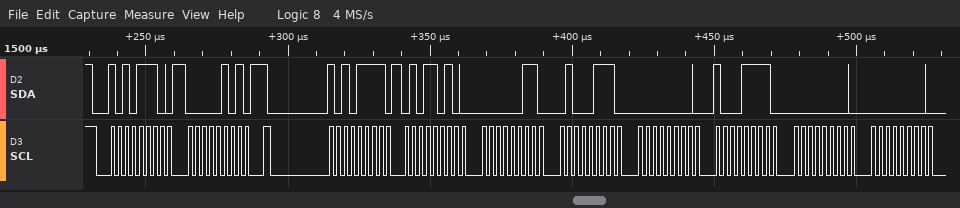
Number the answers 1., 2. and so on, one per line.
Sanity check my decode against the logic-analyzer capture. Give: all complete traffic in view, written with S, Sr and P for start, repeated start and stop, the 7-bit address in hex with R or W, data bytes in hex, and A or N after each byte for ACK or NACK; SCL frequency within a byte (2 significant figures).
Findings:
1. S 57W A 05 A Sr 57R A 5A A 03 A 47 A 00 A 8F A 00 A 00 A
2. 400 kHz
